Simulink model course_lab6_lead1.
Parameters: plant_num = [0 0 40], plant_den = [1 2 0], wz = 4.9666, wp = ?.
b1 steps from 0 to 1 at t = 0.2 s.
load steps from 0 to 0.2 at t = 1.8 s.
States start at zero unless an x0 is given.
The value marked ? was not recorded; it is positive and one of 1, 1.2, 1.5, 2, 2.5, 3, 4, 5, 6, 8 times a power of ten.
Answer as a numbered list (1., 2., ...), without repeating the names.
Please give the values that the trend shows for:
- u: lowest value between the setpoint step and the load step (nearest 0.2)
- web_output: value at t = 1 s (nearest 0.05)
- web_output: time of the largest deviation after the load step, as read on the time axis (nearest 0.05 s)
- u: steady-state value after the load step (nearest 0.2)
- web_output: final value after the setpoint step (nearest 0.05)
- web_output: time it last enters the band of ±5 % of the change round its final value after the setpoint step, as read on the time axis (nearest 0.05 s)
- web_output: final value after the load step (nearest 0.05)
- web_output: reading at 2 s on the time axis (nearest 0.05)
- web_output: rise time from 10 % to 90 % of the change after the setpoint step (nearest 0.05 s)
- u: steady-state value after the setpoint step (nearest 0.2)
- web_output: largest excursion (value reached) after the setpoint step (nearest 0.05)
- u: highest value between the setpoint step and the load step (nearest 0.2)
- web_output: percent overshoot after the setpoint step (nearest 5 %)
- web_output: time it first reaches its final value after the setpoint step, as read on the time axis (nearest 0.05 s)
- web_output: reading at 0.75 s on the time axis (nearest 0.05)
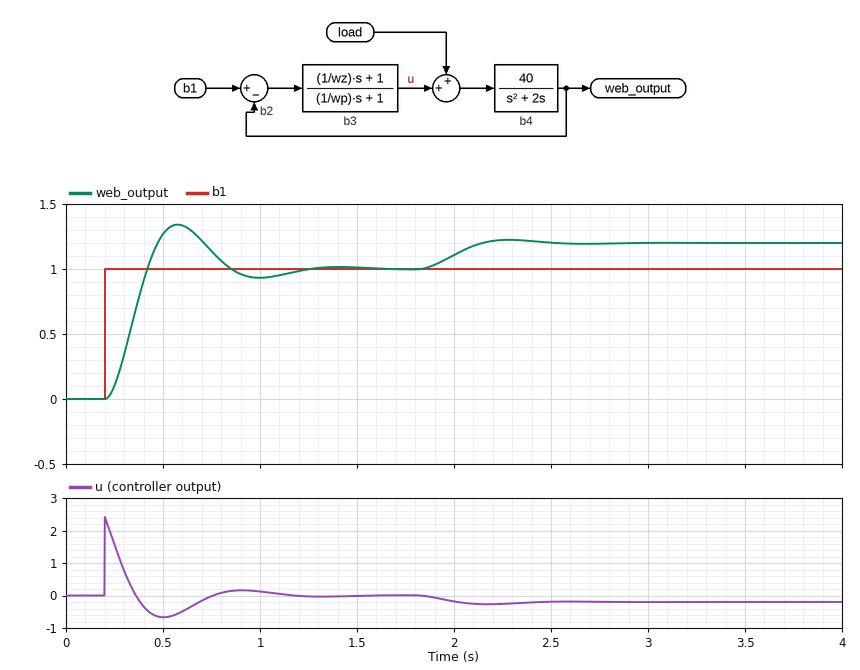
1. -0.6
2. 0.95
3. 2.30 s
4. -0.2
5. 1.00
6. 1.10 s
7. 1.20
8. 1.10
9. 0.15 s
10. 0.0
11. 1.35
12. 2.4
13. 35 %
14. 0.40 s
15. 1.15
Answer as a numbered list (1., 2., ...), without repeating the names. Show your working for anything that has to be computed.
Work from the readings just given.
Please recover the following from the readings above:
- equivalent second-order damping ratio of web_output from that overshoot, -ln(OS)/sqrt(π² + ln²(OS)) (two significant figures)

1. ln(0.35) = -1.050; 1.050 / sqrt(9.870 + 1.102) = 0.32
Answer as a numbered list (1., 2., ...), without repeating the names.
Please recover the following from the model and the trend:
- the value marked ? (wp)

1. 12
